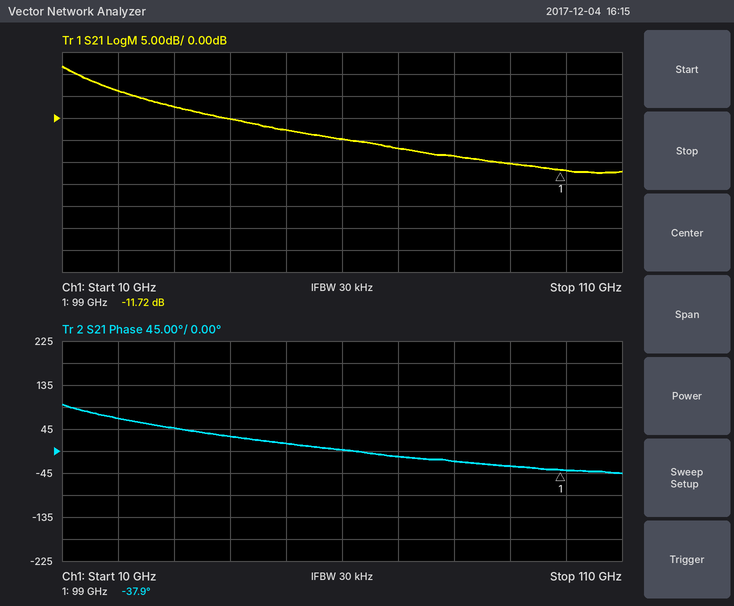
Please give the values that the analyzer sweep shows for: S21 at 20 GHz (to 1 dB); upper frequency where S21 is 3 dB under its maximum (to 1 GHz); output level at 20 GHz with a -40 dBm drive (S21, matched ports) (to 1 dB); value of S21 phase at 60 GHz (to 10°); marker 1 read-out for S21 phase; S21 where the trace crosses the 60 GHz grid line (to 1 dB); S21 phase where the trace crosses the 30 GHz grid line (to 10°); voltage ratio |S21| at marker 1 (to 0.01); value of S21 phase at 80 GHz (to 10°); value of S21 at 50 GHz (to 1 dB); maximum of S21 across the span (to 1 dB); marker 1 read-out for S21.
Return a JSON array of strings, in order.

["6 dB", "15 GHz", "-34 dBm", "0°", "-37.9°", "-5 dB", "50°", "0.26", "-20°", "-3 dB", "12 dB", "-11.72 dB"]
